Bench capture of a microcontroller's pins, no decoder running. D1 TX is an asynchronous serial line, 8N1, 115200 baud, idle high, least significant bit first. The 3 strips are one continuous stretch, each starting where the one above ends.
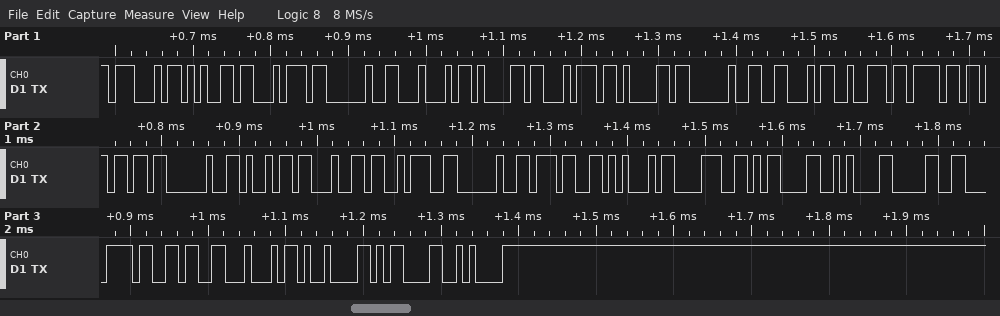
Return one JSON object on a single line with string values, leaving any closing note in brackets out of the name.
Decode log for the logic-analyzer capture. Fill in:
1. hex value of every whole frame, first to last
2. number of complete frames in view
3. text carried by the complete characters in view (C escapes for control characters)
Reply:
{"hex value of every whole frame, first to last": "47 65 74 20 44 61 74 61 20 46 72 6F 6D 20 69 64 3A 20 37 45 38 0D 0A 30 78 36 44 09 0D 0A", "number of complete frames in view": "30", "text carried by the complete characters in view": "\"Get Data From id: 7E8\\r\\n0x6D\\t\\r\\n\""}
